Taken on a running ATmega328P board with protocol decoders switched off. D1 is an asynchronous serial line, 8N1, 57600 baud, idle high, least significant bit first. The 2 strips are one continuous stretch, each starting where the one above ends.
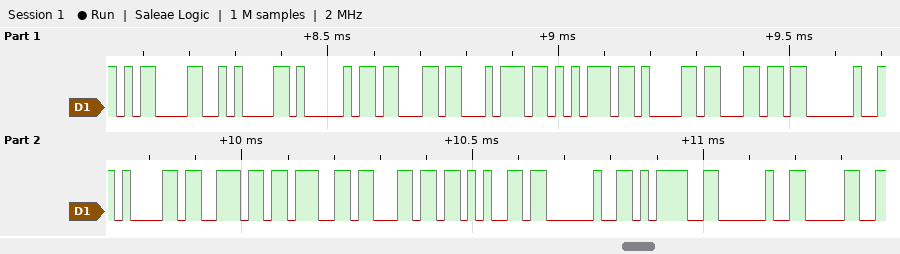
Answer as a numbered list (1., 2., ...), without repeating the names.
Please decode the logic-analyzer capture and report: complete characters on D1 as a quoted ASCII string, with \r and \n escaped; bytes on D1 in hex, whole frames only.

1. "\r\nActual angle = 0"
2. 0D 0A 41 63 74 75 61 6C 20 61 6E 67 6C 65 20 3D 20 30
